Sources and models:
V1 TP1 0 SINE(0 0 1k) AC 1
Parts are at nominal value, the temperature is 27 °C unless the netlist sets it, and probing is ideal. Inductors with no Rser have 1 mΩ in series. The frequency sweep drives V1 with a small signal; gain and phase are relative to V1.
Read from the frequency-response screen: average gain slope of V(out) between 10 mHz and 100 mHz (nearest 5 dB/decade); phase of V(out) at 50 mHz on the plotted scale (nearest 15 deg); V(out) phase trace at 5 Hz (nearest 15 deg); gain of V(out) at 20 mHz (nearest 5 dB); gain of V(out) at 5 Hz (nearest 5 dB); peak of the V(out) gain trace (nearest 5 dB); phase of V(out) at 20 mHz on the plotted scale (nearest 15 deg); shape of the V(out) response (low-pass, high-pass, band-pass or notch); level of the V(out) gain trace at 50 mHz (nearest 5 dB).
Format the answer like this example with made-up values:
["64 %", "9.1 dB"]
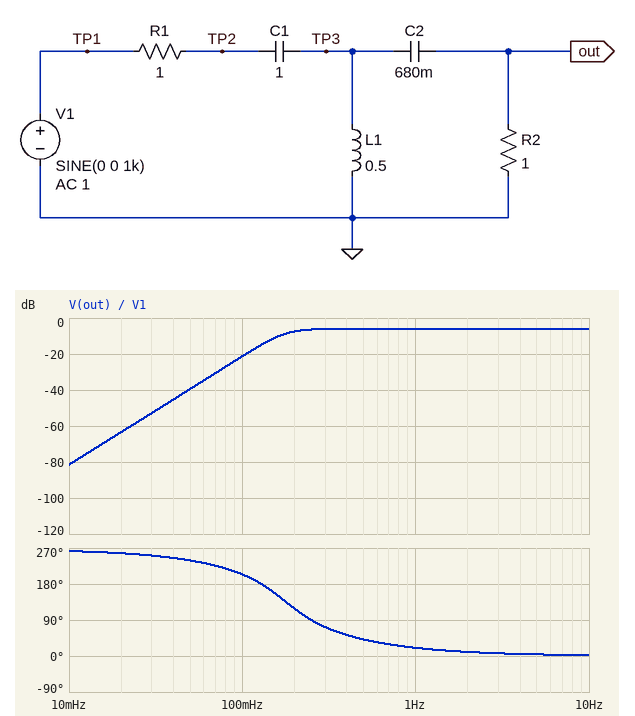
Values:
["60 dB/decade", "240 deg", "0 deg", "-65 dB", "-5 dB", "-5 dB", "255 deg", "high-pass", "-40 dB"]
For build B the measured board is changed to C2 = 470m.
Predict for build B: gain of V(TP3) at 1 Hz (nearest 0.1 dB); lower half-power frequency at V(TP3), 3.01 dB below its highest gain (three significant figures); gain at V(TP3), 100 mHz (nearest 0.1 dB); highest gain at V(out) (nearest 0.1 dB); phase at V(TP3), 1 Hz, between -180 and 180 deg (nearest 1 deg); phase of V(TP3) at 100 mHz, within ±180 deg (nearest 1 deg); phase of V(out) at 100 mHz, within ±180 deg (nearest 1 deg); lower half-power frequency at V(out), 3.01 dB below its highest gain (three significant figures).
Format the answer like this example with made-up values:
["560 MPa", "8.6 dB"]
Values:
["-5.6 dB", "158 mHz", "-13.4 dB", "-6.0 dB", "5 deg", "139 deg", "-147 deg", "197 mHz"]
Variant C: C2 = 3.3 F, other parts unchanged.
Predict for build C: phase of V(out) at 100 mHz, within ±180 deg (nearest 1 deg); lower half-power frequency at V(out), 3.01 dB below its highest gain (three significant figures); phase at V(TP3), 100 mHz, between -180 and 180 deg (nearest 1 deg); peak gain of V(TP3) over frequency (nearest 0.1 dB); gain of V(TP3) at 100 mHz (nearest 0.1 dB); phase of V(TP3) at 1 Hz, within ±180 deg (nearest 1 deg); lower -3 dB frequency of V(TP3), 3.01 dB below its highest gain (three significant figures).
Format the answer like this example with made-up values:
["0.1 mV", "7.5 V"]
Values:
["148 deg", "156 mHz", "123 deg", "-6.0 dB", "-13.7 dB", "12 deg", "148 mHz"]
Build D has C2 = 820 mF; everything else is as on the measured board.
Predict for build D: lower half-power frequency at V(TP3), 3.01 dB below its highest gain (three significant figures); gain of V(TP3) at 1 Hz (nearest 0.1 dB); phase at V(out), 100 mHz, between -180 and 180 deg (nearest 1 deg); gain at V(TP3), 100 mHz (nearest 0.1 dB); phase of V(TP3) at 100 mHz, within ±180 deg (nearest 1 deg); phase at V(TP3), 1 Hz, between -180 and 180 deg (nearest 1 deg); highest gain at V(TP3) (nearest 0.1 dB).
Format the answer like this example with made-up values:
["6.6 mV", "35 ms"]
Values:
["141 mHz", "-5.9 dB", "-162 deg", "-13.0 dB", "136 deg", "8 deg", "-4.2 dB"]
